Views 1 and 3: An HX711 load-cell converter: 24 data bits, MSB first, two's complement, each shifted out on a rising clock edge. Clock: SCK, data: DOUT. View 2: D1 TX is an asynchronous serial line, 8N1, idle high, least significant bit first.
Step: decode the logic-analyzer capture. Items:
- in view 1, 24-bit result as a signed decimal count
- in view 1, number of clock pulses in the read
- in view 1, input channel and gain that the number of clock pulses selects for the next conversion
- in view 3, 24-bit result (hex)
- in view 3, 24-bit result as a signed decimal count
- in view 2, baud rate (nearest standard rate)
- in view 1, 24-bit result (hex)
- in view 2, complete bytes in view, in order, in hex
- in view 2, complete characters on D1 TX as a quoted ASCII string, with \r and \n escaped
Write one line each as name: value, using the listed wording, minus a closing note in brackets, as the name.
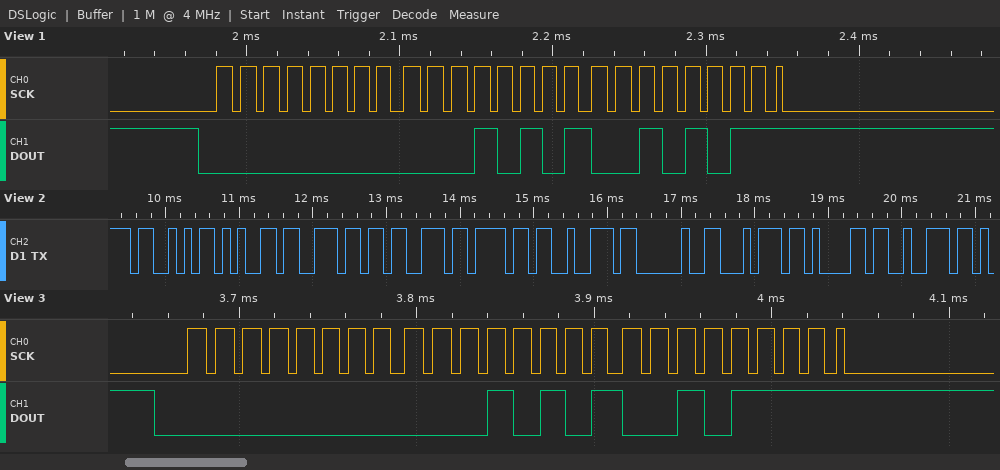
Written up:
in view 1, 24-bit result as a signed decimal count: 5419
in view 1, number of clock pulses in the read: 25
in view 1, input channel and gain that the number of clock pulses selects for the next conversion: channel A, gain 128
in view 3, 24-bit result: 0x00152F
in view 3, 24-bit result as a signed decimal count: 5423
in view 2, baud rate: 9600 baud
in view 1, 24-bit result: 0x00152B
in view 2, complete bytes in view, in order, in hex: 0x53 0x65 0x6E 0x73 0x6F 0x72 0x20 0x74 0x61 0x72
in view 2, complete characters on D1 TX as a quoted ASCII string, with \r and \n escaped: "Sensor tar"
